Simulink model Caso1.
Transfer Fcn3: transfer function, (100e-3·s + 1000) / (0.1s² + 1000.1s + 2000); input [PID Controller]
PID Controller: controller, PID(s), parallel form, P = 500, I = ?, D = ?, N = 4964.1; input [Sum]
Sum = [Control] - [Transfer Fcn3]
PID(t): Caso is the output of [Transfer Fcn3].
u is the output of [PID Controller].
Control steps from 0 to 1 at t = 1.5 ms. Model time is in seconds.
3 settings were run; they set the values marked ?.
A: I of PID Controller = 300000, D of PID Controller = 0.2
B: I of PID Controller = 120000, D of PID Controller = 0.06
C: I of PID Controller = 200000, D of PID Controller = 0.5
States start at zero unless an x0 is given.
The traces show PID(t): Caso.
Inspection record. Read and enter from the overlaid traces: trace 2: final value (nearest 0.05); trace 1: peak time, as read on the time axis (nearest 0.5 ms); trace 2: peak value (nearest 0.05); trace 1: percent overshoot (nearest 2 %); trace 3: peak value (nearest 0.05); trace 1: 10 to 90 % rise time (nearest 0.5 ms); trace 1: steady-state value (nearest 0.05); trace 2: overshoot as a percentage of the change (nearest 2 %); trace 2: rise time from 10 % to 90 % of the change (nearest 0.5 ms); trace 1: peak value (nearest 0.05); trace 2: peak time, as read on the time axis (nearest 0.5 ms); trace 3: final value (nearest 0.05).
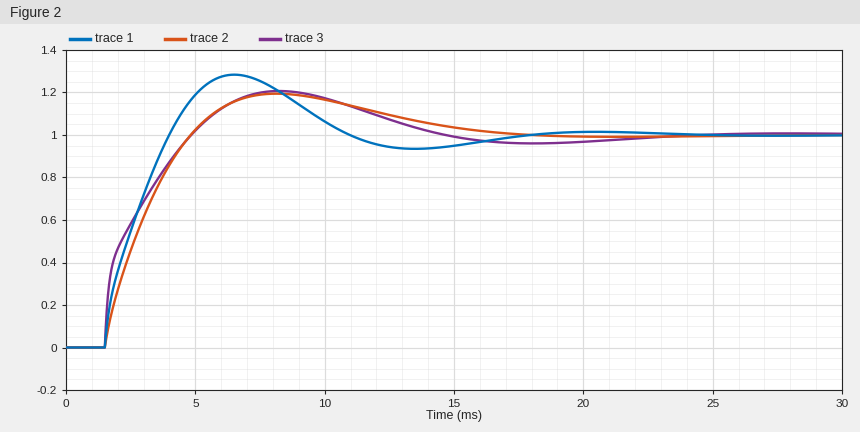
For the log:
1.00
6.5 ms
1.20
28 %
1.20
2.0 ms
1.00
20 %
2.5 ms
1.30
8.0 ms
1.00
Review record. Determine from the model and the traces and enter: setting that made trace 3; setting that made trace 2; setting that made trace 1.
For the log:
C
B
A
